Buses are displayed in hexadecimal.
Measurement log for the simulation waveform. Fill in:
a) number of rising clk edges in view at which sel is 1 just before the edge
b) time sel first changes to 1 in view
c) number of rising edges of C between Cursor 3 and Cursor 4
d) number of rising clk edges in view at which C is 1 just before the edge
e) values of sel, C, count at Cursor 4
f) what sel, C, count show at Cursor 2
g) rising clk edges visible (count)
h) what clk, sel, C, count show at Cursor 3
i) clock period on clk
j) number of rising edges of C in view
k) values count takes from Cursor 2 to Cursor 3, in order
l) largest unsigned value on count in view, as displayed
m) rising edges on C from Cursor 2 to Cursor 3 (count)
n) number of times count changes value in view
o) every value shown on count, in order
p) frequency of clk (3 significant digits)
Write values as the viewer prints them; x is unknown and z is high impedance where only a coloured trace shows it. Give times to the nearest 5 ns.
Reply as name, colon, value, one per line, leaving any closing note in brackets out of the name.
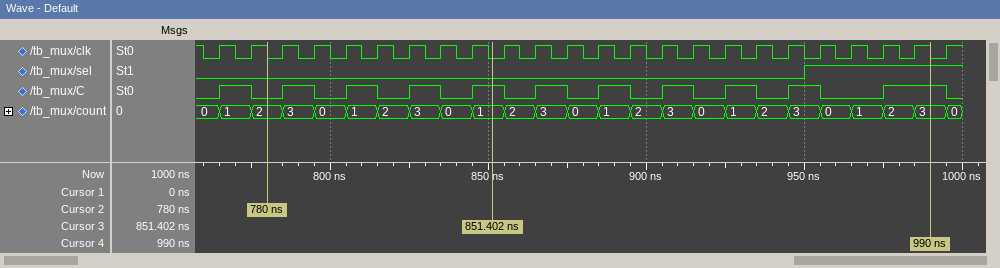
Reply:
number of rising clk edges in view at which sel is 1 just before the edge: 5
time sel first changes to 1 in view: 950 ns
number of rising edges of C between Cursor 3 and Cursor 4: 6
number of rising clk edges in view at which C is 1 just before the edge: 12
values of sel, C, count at Cursor 4: sel=1, C=1, count=3
what sel, C, count show at Cursor 2: sel=0, C=0, count=2
rising clk edges visible: 24
what clk, sel, C, count show at Cursor 3: clk=0, sel=0, C=1, count=1
clock period on clk: 10 ns
number of rising edges of C in view: 11
values count takes from Cursor 2 to Cursor 3, in order: 2, 3, 0, 1, 2, 3, 0, 1
largest unsigned value on count in view, as displayed: 3
rising edges on C from Cursor 2 to Cursor 3: 4
number of times count changes value in view: 24
every value shown on count, in order: 0, 1, 2, 3, 0, 1, 2, 3, 0, 1, 2, 3, 0, 1, 2, 3, 0, 1, 2, 3, 0, 1, 2, 3, 0
frequency of clk: 100 MHz
